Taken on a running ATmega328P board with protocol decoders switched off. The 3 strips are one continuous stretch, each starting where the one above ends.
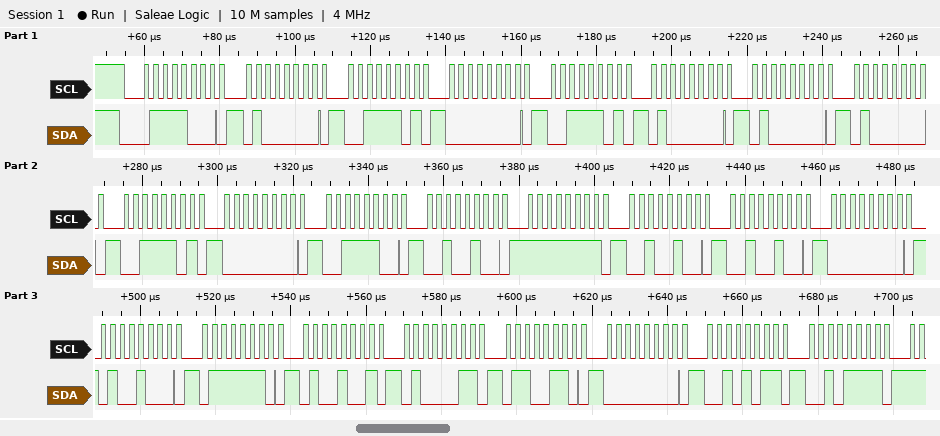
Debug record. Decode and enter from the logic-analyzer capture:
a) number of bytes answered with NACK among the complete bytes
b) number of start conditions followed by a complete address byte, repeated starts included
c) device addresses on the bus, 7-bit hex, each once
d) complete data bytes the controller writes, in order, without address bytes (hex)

0
1
0x3C
40 3D 00 3D 40 40 40 3D 00 3C 24 FF 24 24 00 48 7E 49 43 66 00 2B 2F
